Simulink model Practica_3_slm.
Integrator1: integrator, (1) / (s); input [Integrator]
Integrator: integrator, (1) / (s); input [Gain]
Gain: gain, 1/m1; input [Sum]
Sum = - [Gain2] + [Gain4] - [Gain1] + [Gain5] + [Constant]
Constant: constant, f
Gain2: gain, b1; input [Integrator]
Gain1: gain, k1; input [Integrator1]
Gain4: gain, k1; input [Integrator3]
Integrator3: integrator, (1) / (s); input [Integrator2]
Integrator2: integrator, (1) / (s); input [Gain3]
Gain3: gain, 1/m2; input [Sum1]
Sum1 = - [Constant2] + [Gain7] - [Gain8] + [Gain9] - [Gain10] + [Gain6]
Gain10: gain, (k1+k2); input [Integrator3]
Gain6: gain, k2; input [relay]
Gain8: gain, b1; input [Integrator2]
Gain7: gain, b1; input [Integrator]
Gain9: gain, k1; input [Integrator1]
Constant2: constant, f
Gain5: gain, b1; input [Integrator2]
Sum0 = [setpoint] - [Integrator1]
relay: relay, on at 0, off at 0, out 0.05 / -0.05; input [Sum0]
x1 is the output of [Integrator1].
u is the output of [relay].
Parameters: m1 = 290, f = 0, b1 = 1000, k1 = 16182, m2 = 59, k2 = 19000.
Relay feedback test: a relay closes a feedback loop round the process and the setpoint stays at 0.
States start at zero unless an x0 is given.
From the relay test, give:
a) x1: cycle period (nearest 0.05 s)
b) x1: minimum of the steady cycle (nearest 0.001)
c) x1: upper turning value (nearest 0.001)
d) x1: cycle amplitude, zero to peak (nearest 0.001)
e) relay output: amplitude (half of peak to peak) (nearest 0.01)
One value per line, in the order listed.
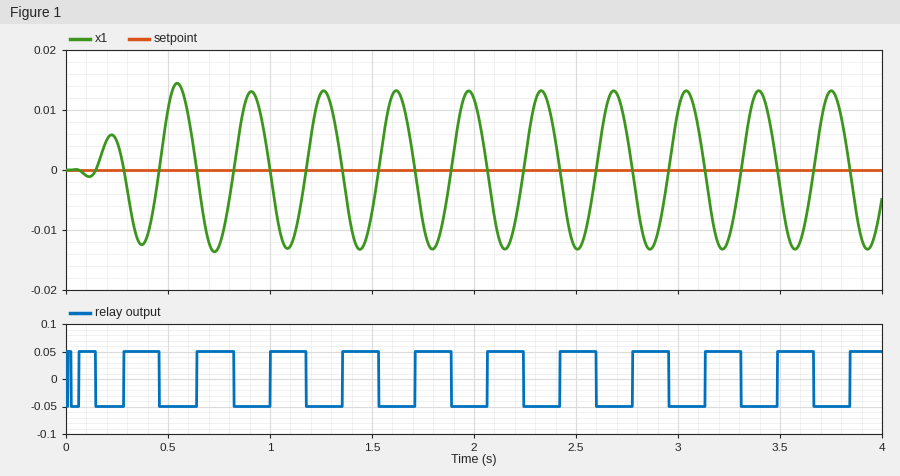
0.35 s
-0.013
0.013
0.013
0.05
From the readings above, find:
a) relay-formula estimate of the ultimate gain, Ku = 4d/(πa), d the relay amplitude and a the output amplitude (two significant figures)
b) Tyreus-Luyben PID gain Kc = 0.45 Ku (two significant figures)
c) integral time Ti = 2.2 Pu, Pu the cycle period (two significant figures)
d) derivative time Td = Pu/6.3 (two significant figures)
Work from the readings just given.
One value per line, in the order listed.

4.9
2.2
0.77 s
0.056 s
